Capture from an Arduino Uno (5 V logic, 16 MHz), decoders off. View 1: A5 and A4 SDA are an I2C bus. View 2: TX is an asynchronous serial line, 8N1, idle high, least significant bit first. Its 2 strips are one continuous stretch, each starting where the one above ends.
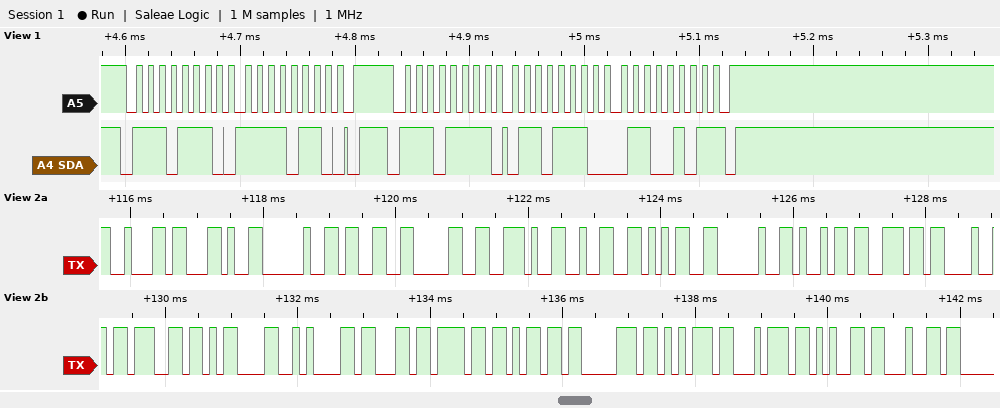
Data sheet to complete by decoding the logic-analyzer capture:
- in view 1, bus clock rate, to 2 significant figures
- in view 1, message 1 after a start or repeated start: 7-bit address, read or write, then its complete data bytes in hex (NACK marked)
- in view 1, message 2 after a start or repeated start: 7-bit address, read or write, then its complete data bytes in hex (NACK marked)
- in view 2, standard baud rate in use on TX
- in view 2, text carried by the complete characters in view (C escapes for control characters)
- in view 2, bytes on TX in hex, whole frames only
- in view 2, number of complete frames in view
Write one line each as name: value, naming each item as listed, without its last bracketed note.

in view 1, bus clock rate, to 2 significant figures: 100 kHz
in view 1, message 1 after a start or repeated start: 7-bit address, read or write, then its complete data bytes in hex: 0x77 write: F6
in view 1, message 2 after a start or repeated start: 7-bit address, read or write, then its complete data bytes in hex: 0x77 read: 6E 65 NACK
in view 2, standard baud rate in use on TX: 9600 baud
in view 2, text carried by the complete characters in view: "b, 30.25 inHg\r\ncomputed"
in view 2, bytes on TX in hex, whole frames only: 0x62 0x2C 0x20 0x33 0x30 0x2E 0x32 0x35 0x20 0x69 0x6E 0x48 0x67 0x0D 0x0A 0x63 0x6F 0x6D 0x70 0x75 0x74 0x65 0x64
in view 2, number of complete frames in view: 23
